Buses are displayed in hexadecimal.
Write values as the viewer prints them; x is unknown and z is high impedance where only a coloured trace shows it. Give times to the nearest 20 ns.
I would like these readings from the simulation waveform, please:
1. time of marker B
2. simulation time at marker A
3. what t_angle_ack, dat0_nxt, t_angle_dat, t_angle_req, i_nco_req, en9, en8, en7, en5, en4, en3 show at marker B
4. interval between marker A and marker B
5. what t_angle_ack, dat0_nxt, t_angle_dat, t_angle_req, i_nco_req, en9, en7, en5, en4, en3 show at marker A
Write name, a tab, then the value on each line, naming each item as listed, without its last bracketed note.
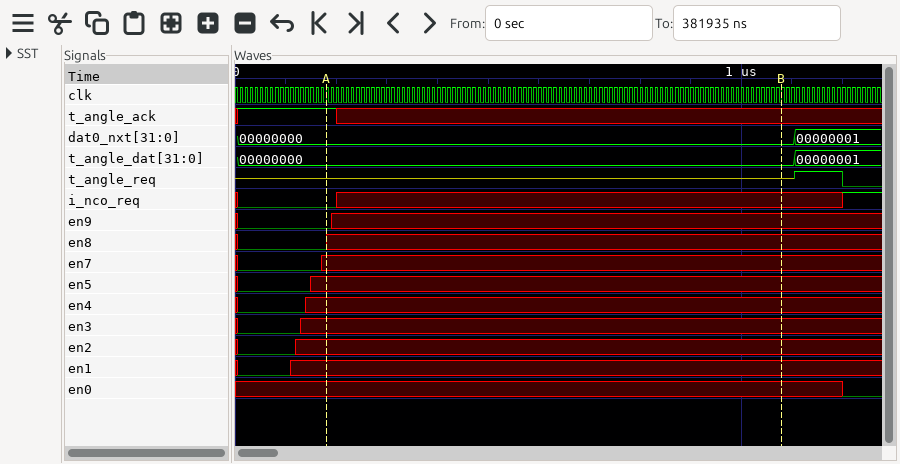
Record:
time of marker B	1080 ns
simulation time at marker A	180 ns
what t_angle_ack, dat0_nxt, t_angle_dat, t_angle_req, i_nco_req, en9, en8, en7, en5, en4, en3 show at marker B	t_angle_ack=x, dat0_nxt=00000000, t_angle_dat=00000000, t_angle_req=z, i_nco_req=x, en9=x, en8=x, en7=x, en5=x, en4=x, en3=x
interval between marker A and marker B	900 ns
what t_angle_ack, dat0_nxt, t_angle_dat, t_angle_req, i_nco_req, en9, en7, en5, en4, en3 show at marker A	t_angle_ack=1, dat0_nxt=00000000, t_angle_dat=00000000, t_angle_req=z, i_nco_req=0, en9=0, en7=x, en5=x, en4=x, en3=x
